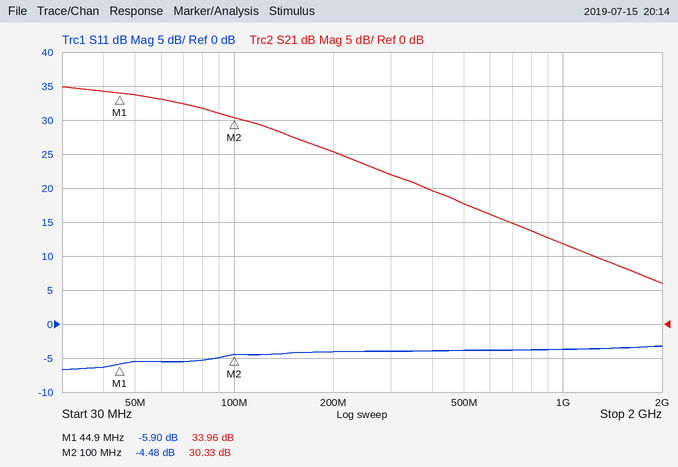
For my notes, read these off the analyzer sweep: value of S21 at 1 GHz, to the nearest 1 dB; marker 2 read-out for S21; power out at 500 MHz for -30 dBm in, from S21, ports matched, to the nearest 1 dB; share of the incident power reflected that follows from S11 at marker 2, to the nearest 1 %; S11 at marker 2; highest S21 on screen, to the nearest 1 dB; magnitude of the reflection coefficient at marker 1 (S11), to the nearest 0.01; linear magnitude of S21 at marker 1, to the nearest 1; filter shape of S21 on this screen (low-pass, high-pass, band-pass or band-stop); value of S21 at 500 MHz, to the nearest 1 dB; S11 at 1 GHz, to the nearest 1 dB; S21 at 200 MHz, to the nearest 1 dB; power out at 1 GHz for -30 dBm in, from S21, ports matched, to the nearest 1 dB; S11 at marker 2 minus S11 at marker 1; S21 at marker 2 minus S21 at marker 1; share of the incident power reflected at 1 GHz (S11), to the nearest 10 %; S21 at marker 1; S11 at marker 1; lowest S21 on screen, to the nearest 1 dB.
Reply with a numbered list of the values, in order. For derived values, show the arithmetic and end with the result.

1. 12 dB
2. 30.33 dB
3. -30 dBm + (18 dB) = -12 dBm
4. 10^(-4.48/10) ≈ 36 %
5. -4.48 dB
6. 35 dB
7. 10^(-5.9/20) ≈ 0.51
8. 10^(33.96/20) ≈ 50
9. low-pass
10. 18 dB
11. -4 dB
12. 25 dB
13. -30 dBm + (12 dB) = -18 dBm
14. -4.48 − (-5.9) = 1.42 dB
15. 30.33 − (33.96) = -3.63 dB
16. 10^(-4/10) ≈ 40 %
17. 33.96 dB
18. -5.90 dB
19. 6 dB
